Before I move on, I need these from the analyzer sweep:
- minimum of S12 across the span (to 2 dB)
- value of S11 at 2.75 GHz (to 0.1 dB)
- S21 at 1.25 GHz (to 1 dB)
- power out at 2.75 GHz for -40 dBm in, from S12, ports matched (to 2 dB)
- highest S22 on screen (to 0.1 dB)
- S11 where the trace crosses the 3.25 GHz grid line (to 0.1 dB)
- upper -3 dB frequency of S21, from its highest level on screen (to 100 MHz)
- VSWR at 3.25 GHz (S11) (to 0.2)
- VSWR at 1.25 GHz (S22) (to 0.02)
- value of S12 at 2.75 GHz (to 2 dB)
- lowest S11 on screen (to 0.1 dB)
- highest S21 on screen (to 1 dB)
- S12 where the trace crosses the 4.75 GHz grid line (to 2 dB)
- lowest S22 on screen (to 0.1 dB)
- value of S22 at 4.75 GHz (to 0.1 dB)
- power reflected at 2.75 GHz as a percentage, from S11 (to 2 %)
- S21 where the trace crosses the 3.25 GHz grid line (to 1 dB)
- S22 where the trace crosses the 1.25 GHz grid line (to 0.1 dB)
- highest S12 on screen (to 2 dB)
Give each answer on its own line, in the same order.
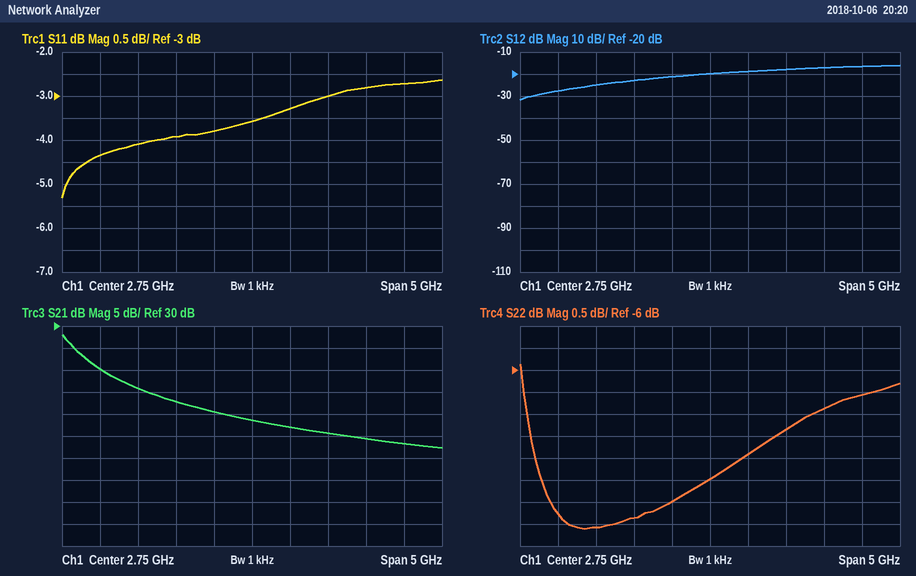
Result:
-32 dB
-3.6 dB
16 dB
-60 dBm
-5.9 dB
-3.3 dB
400 MHz
5.4
2.00
-20 dB
-5.3 dB
28 dB
-16 dB
-9.6 dB
-6.6 dB
44 %
7 dB
-9.6 dB
-16 dB
